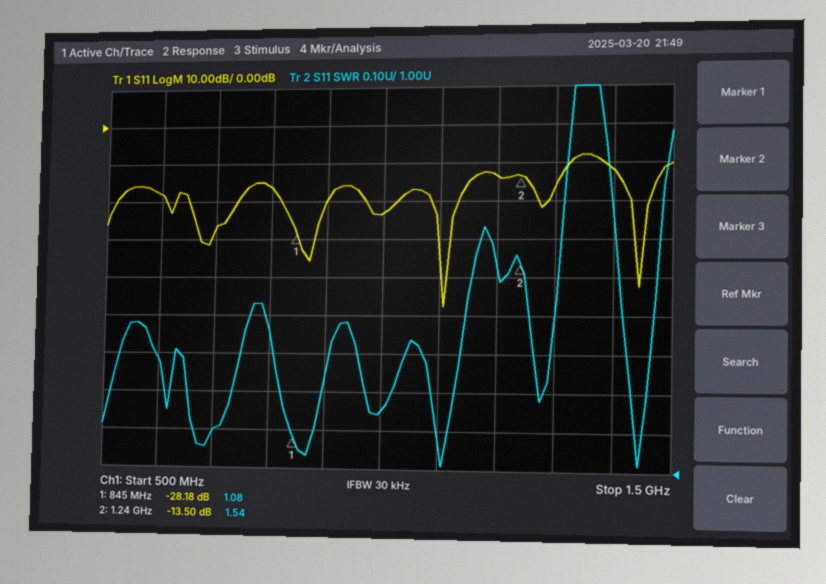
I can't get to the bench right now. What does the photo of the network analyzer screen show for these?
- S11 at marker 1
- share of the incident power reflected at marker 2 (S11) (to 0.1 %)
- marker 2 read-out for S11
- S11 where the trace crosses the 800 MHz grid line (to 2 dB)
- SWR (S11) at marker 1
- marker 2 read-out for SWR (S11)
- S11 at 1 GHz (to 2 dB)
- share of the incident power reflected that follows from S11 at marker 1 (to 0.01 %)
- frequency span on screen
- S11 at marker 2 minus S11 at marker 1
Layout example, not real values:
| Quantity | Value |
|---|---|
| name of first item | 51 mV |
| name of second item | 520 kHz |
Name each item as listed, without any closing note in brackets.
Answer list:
| Quantity | Value |
|---|---|
| S11 at marker 1 | -28.18 dB |
| share of the incident power reflected at marker 2 (S11) | 4.5 % |
| marker 2 read-out for S11 | -13.50 dB |
| S11 where the trace crosses the 800 MHz grid line | -16 dB |
| SWR (S11) at marker 1 | 1.08 |
| marker 2 read-out for SWR | 1.54 |
| S11 at 1 GHz | -24 dB |
| share of the incident power reflected that follows from S11 at marker 1 | 0.15 % |
| frequency span on screen | 1 GHz |
| S11 at marker 2 minus S11 at marker 1 | 14.68 dB |
